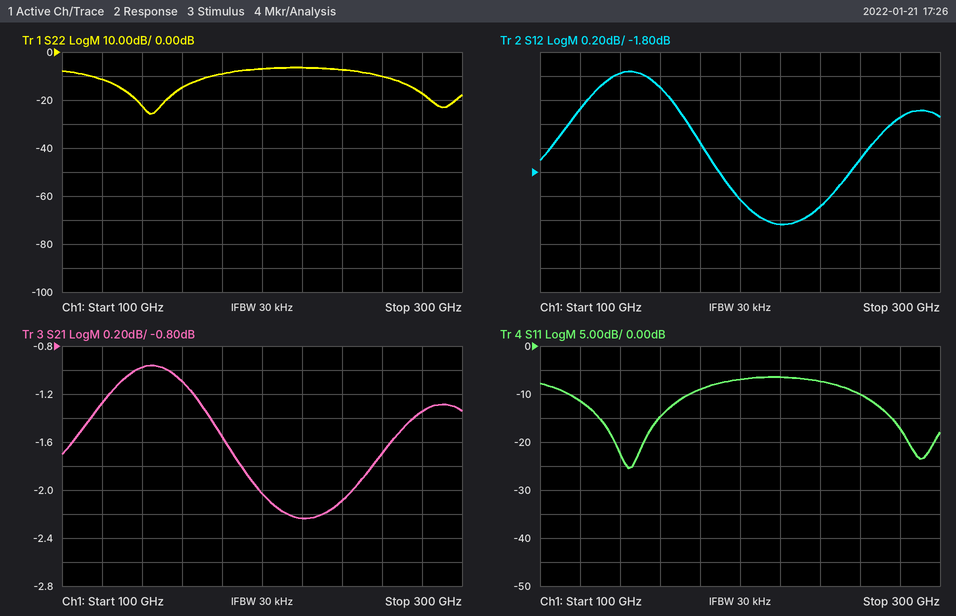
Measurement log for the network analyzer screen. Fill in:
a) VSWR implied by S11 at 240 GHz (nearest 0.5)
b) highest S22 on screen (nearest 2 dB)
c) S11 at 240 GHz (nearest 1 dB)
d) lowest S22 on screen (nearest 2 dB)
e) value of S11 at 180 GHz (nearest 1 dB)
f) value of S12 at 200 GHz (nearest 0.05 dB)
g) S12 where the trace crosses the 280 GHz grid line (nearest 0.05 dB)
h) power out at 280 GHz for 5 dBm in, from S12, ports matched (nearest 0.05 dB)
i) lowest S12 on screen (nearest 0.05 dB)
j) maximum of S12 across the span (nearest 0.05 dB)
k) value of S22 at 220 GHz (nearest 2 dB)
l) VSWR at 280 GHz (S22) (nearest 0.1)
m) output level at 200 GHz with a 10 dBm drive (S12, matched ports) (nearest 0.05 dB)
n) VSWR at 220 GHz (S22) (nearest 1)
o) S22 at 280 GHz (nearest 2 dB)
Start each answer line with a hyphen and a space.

- 2.5
- -6 dB
- -7 dB
- -26 dB
- -9 dB
- -2.05 dB
- -1.35 dB
- 3.65 dBm
- -2.25 dB
- -0.95 dB
- -6 dB
- 1.3
- 7.95 dBm
- 3
- -18 dB
